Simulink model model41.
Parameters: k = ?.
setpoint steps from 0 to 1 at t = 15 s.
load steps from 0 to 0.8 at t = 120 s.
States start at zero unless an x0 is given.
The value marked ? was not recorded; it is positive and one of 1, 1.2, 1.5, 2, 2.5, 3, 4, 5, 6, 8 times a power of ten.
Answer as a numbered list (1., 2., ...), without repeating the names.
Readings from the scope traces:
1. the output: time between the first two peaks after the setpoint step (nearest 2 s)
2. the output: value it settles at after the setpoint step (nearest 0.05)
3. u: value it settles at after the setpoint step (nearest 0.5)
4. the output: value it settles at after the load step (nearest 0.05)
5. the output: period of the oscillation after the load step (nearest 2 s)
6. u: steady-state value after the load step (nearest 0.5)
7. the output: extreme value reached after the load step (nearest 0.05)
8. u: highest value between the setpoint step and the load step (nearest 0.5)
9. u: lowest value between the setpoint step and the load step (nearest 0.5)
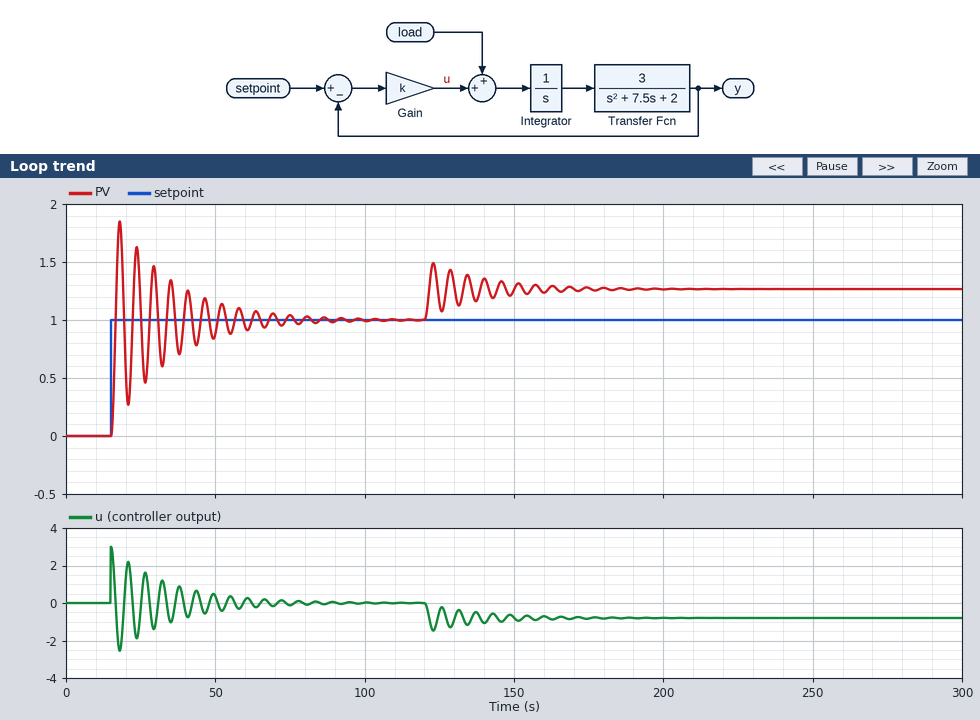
1. 6 s
2. 1.00
3. 0.0
4. 1.25
5. 6 s
6. -1.0
7. 1.50
8. 3.0
9. -2.5
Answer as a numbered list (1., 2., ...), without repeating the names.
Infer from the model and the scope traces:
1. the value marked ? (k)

1. 3
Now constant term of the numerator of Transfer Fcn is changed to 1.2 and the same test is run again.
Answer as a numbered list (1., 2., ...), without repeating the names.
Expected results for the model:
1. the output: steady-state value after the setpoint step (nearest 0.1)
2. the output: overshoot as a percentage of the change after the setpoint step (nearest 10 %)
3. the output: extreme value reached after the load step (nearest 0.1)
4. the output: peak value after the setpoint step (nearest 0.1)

1. 1.0
2. 60 %
3. 1.4
4. 1.6
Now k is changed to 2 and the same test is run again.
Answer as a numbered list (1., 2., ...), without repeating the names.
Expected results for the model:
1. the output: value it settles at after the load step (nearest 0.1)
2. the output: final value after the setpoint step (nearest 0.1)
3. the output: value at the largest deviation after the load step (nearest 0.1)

1. 1.4
2. 1.0
3. 1.7
